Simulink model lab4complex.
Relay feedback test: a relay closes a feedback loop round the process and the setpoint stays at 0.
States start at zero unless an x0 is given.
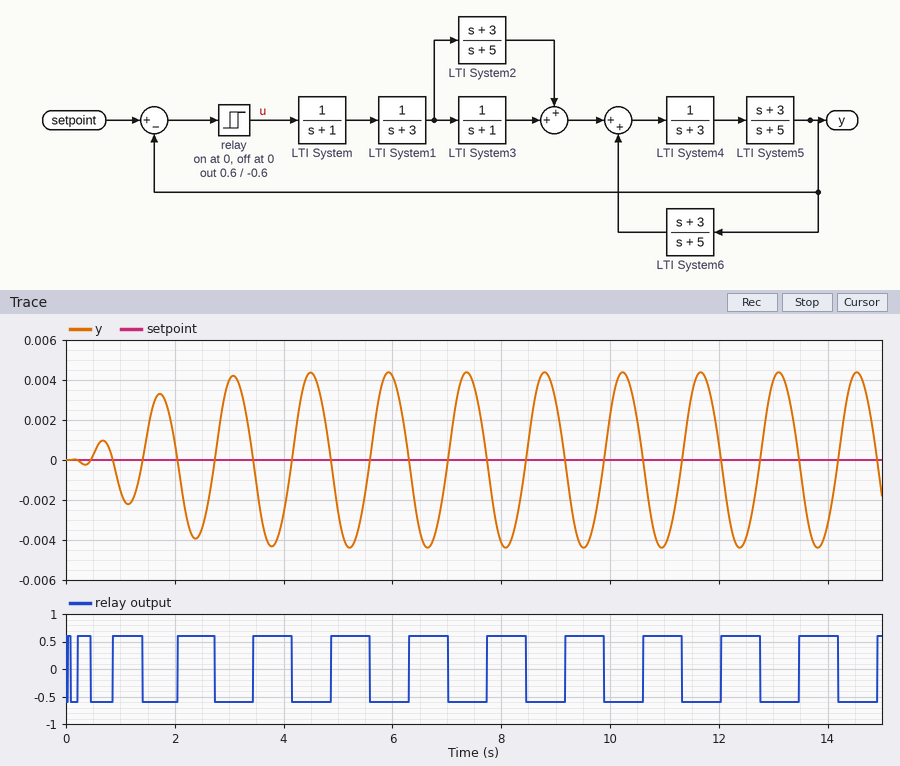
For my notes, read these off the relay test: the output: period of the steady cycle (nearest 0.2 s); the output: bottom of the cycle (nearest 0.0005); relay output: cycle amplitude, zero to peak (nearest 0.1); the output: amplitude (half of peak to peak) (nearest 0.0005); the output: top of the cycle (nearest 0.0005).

1.4 s
-0.0045
0.6
0.0045
0.0045
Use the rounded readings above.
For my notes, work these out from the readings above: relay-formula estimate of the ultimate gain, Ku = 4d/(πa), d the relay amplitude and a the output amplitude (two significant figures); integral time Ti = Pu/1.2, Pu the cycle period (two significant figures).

170
1.2 s
